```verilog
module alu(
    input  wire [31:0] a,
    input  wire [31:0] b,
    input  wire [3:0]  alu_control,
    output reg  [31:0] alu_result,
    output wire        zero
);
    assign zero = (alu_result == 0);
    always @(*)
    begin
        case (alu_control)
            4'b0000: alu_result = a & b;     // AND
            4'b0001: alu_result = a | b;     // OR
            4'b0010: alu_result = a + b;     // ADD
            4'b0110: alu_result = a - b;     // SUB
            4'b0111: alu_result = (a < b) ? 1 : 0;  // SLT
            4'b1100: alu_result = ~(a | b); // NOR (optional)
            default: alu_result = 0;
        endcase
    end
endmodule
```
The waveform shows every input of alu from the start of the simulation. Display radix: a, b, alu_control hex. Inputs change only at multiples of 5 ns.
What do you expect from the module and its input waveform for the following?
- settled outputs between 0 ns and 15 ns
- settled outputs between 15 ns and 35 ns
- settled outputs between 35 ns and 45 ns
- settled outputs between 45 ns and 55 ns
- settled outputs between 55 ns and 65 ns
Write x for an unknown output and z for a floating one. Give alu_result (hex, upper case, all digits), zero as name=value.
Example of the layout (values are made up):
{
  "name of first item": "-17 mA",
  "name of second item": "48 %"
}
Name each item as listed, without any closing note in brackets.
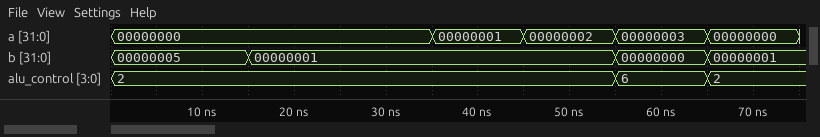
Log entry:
{
  "settled outputs between 0 ns and 15 ns": "alu_result=00000005, zero=0",
  "settled outputs between 15 ns and 35 ns": "alu_result=00000001, zero=0",
  "settled outputs between 35 ns and 45 ns": "alu_result=00000002, zero=0",
  "settled outputs between 45 ns and 55 ns": "alu_result=00000003, zero=0",
  "settled outputs between 55 ns and 65 ns": "alu_result=00000003, zero=0"
}
